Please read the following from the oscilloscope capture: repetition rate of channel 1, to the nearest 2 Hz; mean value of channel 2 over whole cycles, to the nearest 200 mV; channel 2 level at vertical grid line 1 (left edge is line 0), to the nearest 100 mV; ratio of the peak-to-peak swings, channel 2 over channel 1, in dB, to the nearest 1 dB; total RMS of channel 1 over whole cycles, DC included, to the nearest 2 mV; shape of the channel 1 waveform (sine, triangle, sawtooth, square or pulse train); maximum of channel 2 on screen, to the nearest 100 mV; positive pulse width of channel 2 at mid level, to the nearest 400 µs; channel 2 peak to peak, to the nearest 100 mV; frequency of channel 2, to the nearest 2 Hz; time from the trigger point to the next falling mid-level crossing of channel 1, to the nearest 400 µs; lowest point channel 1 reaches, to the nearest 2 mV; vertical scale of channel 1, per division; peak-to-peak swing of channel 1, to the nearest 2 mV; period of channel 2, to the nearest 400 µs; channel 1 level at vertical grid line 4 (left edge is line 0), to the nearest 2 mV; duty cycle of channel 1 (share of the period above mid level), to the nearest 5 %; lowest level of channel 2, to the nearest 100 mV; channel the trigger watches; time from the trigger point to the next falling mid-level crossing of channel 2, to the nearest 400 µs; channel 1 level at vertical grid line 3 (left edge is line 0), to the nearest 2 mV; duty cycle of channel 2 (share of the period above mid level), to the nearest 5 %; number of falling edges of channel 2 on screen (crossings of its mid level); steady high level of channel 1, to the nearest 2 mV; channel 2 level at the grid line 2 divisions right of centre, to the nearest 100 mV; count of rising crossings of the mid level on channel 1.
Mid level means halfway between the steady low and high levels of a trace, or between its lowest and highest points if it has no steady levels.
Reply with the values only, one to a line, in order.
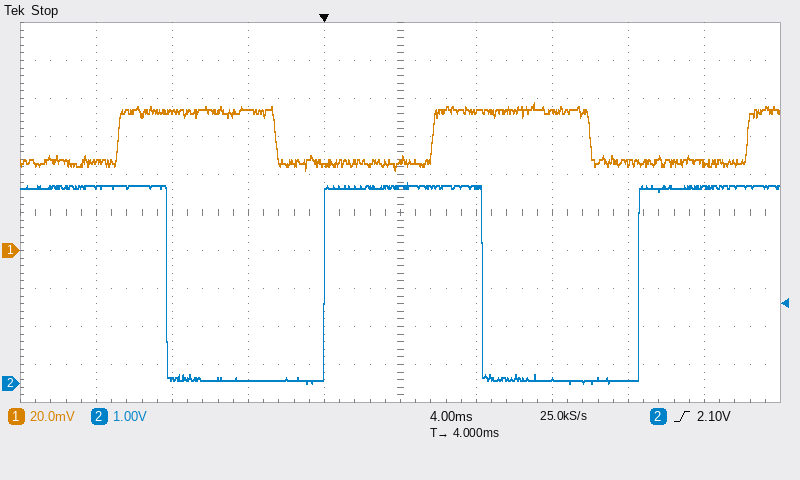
60 Hz
2.6 V
5.2 V
43 dB
62 mV
square
5.3 V
8.4 ms
5.3 V
60 Hz
14.0 ms
42 mV
20 mV
36 mV
16.4 ms
46 mV
50 %
0.0 V
channel 2
8.4 ms
74 mV
50 %
2
74 mV
100 mV
3
